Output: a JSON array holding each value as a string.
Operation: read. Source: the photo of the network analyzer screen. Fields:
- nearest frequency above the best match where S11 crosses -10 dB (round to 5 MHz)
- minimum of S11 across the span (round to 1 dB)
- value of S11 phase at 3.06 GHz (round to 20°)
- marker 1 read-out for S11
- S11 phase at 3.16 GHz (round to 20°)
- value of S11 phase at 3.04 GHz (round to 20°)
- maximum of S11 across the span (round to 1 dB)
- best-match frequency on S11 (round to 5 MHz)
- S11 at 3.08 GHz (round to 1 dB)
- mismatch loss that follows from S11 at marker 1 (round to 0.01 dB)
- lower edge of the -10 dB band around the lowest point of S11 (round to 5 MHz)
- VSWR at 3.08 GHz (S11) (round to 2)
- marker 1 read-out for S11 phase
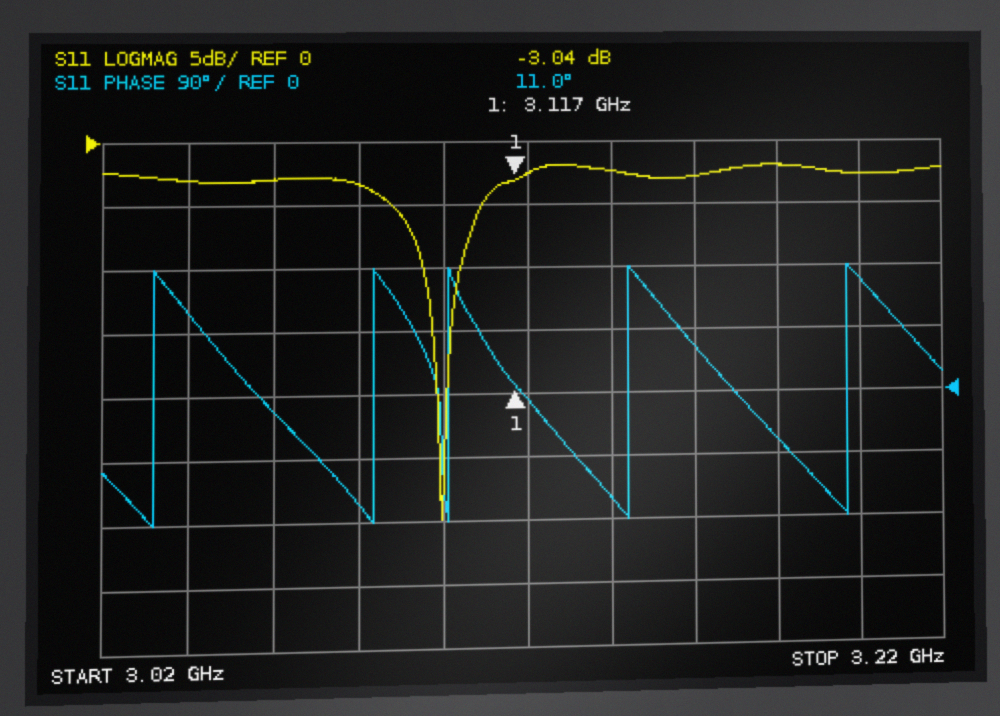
["3.105 GHz", "-30 dB", "-20°", "-3.04 dB", "60°", "120°", "-2 dB", "3.100 GHz", "-3 dB", "2.98 dB", "3.095 GHz", "6", "11.0°"]
